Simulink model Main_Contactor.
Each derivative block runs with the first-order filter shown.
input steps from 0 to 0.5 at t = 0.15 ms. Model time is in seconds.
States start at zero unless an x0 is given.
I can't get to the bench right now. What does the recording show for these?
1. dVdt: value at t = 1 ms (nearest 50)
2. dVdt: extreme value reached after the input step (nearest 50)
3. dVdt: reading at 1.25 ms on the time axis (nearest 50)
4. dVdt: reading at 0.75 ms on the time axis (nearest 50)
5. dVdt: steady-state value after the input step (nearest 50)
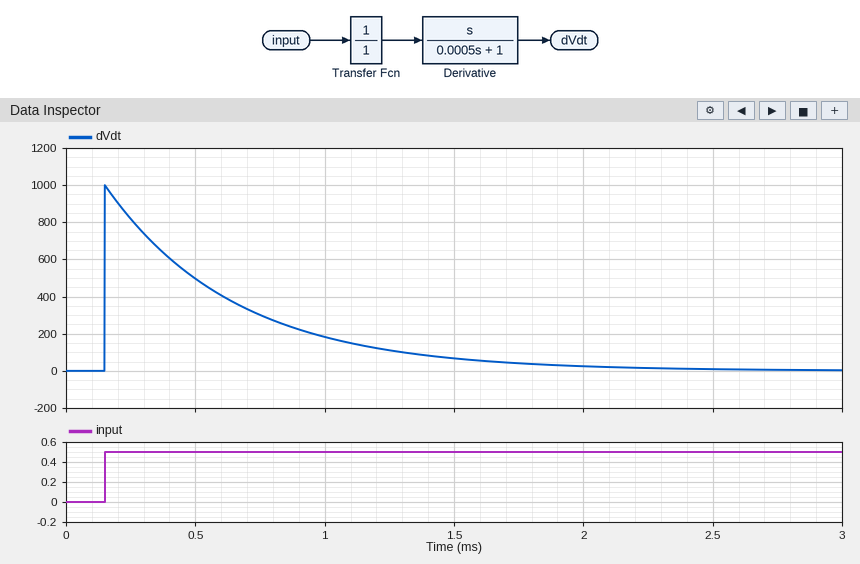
200
1000
100
300
0
